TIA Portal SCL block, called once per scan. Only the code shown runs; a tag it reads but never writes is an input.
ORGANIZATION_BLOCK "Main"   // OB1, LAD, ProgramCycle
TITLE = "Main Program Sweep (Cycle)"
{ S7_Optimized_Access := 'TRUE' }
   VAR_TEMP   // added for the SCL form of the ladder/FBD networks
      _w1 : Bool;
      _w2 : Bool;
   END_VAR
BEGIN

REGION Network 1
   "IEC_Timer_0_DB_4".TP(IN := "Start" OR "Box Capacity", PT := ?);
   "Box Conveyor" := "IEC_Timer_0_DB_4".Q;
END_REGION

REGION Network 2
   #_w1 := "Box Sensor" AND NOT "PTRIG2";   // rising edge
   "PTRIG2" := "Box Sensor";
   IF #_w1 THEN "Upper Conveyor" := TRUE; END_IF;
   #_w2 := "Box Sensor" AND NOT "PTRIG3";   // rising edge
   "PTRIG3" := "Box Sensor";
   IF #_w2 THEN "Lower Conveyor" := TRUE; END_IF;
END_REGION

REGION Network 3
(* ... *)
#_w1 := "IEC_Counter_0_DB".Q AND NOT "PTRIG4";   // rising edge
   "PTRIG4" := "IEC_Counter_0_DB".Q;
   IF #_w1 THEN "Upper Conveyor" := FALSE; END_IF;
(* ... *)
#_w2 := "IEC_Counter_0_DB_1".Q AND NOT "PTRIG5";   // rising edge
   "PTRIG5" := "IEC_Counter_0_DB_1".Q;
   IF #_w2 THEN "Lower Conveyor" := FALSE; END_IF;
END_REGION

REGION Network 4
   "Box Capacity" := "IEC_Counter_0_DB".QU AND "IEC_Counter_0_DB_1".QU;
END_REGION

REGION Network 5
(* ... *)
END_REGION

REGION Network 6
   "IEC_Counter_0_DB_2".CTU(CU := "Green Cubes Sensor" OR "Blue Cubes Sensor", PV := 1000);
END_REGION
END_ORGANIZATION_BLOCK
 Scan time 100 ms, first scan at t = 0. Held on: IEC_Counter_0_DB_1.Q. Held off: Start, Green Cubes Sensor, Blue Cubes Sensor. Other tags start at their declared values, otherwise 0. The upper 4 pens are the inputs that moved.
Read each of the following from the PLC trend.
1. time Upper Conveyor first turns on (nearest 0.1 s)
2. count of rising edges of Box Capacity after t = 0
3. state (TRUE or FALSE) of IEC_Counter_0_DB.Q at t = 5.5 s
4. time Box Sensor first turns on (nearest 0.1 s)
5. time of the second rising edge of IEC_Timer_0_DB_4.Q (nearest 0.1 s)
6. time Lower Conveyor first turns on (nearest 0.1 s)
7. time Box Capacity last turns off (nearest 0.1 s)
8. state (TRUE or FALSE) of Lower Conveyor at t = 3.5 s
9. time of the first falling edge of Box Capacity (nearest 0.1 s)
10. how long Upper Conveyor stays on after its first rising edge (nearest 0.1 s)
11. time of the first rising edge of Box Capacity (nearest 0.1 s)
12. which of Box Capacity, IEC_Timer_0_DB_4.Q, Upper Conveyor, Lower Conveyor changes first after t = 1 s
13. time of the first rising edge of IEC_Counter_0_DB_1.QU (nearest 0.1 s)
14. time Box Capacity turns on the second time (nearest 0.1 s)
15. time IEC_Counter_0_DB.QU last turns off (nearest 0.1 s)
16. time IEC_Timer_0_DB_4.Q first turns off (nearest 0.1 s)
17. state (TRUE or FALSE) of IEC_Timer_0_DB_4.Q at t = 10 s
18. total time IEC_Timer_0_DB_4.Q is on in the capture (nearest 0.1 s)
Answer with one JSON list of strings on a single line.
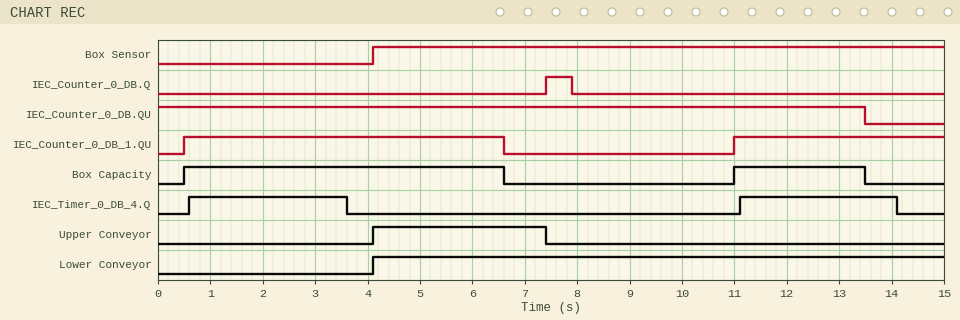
["4.1 s", "2", "FALSE", "4.1 s", "11.1 s", "4.1 s", "13.5 s", "FALSE", "6.6 s", "3.3 s", "0.5 s", "IEC_Timer_0_DB_4.Q", "0.5 s", "11.0 s", "13.5 s", "3.6 s", "FALSE", "6.0 s"]
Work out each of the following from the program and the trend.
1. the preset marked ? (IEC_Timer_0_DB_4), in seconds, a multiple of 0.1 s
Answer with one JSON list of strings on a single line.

["3.0 s"]
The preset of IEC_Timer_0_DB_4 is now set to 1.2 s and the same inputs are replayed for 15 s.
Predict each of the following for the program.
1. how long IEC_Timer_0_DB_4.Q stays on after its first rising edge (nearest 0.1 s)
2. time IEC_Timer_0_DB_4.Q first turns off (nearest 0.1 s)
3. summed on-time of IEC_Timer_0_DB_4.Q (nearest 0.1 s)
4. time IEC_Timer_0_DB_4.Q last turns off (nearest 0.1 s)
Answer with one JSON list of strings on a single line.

["1.2 s", "1.8 s", "2.4 s", "12.3 s"]
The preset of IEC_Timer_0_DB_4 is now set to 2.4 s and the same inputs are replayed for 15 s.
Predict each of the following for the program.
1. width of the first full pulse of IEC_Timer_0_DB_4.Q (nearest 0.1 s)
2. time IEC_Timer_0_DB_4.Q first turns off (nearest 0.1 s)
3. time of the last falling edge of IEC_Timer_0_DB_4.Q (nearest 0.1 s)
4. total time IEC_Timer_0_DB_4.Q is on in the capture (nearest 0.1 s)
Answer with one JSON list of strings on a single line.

["2.4 s", "3.0 s", "13.5 s", "4.8 s"]
